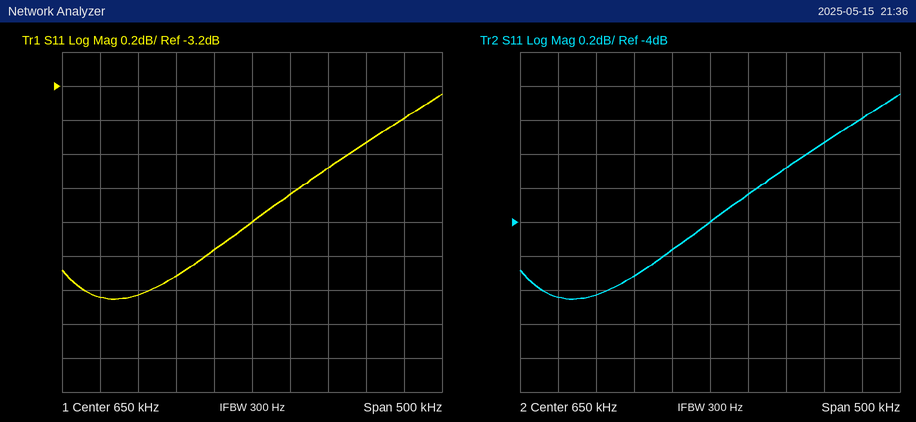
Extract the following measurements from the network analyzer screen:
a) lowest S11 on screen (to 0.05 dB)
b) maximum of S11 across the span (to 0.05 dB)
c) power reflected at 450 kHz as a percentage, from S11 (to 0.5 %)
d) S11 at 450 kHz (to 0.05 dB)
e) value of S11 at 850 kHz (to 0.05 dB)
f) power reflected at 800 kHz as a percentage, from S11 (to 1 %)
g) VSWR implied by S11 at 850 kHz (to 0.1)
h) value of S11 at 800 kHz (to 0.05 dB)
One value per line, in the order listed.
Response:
-4.45 dB
-3.25 dB
36.0 %
-4.45 dB
-3.40 dB
44 %
5.2
-3.55 dB
